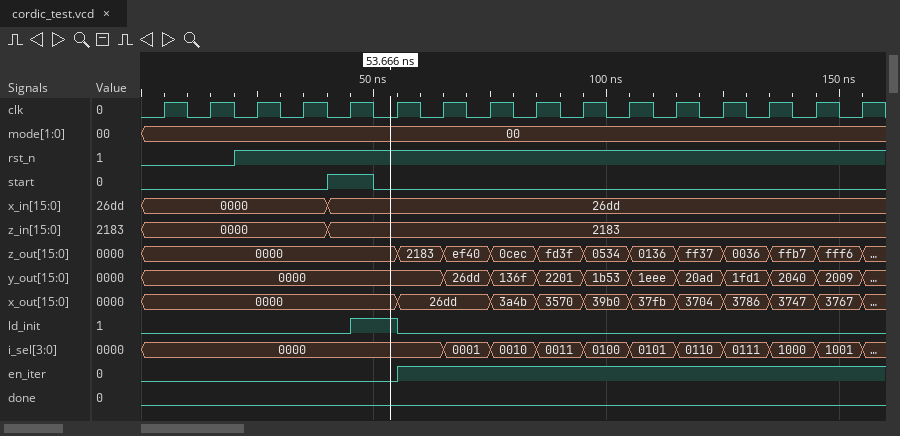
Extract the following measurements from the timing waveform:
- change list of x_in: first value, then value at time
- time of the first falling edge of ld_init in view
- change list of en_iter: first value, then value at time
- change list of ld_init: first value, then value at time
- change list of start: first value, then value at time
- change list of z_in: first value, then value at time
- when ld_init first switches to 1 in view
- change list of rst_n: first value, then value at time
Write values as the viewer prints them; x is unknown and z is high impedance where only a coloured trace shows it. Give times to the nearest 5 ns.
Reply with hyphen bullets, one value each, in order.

- 0000, 26dd at 40 ns
- 55 ns
- 0, 1 at 55 ns
- 0, 1 at 45 ns, 0 at 55 ns
- 0, 1 at 40 ns, 0 at 50 ns
- 0000, 2183 at 40 ns
- 45 ns
- 0, 1 at 20 ns
